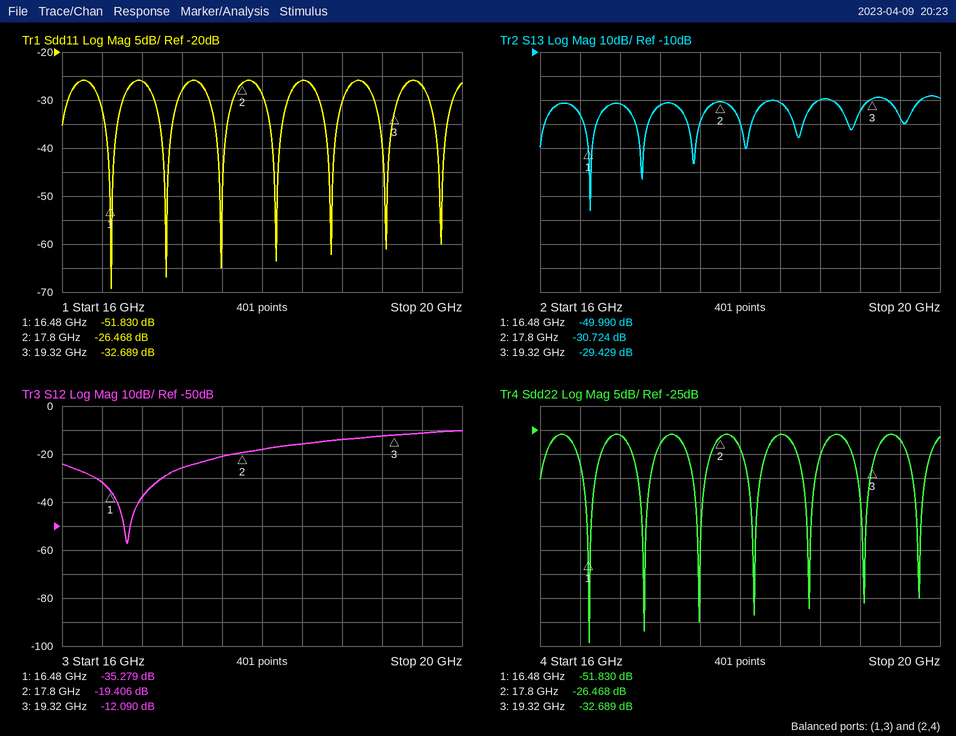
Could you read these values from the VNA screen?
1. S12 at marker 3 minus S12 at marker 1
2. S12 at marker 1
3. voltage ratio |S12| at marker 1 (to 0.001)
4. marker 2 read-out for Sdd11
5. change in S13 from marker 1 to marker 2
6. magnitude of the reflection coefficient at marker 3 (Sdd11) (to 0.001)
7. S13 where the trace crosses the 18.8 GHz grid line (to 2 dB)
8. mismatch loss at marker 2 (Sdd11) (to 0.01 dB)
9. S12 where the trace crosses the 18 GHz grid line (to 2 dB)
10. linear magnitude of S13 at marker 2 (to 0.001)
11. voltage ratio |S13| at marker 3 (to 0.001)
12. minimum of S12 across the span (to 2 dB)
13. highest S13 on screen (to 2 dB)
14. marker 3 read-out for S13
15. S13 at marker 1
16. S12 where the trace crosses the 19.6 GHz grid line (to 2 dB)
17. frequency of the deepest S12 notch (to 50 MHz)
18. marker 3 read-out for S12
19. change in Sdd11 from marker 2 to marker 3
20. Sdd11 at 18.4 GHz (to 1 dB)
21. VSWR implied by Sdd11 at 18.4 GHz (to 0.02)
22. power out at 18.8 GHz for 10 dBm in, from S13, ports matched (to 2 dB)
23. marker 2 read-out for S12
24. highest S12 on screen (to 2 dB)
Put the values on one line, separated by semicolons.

23.189 dB; -35.279 dB; 0.017; -26.468 dB; 19.266 dB; 0.023; -30 dB; 0.01 dB; -18 dB; 0.029; 0.034; -58 dB; -28 dB; -29.429 dB; -49.990 dB; -12 dB; 16.65 GHz; -12.090 dB; -6.221 dB; -26 dB; 1.10; -20 dBm; -19.406 dB; -10 dB
